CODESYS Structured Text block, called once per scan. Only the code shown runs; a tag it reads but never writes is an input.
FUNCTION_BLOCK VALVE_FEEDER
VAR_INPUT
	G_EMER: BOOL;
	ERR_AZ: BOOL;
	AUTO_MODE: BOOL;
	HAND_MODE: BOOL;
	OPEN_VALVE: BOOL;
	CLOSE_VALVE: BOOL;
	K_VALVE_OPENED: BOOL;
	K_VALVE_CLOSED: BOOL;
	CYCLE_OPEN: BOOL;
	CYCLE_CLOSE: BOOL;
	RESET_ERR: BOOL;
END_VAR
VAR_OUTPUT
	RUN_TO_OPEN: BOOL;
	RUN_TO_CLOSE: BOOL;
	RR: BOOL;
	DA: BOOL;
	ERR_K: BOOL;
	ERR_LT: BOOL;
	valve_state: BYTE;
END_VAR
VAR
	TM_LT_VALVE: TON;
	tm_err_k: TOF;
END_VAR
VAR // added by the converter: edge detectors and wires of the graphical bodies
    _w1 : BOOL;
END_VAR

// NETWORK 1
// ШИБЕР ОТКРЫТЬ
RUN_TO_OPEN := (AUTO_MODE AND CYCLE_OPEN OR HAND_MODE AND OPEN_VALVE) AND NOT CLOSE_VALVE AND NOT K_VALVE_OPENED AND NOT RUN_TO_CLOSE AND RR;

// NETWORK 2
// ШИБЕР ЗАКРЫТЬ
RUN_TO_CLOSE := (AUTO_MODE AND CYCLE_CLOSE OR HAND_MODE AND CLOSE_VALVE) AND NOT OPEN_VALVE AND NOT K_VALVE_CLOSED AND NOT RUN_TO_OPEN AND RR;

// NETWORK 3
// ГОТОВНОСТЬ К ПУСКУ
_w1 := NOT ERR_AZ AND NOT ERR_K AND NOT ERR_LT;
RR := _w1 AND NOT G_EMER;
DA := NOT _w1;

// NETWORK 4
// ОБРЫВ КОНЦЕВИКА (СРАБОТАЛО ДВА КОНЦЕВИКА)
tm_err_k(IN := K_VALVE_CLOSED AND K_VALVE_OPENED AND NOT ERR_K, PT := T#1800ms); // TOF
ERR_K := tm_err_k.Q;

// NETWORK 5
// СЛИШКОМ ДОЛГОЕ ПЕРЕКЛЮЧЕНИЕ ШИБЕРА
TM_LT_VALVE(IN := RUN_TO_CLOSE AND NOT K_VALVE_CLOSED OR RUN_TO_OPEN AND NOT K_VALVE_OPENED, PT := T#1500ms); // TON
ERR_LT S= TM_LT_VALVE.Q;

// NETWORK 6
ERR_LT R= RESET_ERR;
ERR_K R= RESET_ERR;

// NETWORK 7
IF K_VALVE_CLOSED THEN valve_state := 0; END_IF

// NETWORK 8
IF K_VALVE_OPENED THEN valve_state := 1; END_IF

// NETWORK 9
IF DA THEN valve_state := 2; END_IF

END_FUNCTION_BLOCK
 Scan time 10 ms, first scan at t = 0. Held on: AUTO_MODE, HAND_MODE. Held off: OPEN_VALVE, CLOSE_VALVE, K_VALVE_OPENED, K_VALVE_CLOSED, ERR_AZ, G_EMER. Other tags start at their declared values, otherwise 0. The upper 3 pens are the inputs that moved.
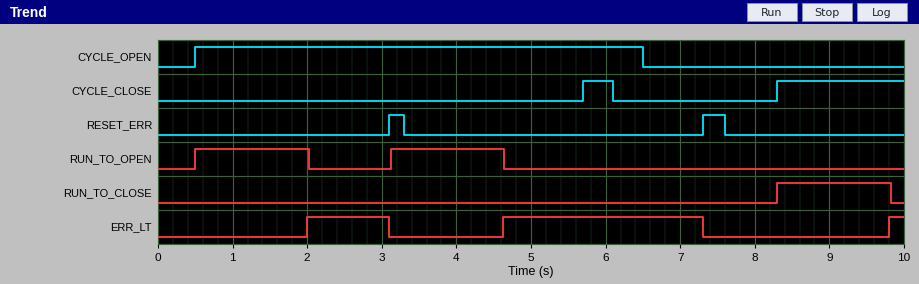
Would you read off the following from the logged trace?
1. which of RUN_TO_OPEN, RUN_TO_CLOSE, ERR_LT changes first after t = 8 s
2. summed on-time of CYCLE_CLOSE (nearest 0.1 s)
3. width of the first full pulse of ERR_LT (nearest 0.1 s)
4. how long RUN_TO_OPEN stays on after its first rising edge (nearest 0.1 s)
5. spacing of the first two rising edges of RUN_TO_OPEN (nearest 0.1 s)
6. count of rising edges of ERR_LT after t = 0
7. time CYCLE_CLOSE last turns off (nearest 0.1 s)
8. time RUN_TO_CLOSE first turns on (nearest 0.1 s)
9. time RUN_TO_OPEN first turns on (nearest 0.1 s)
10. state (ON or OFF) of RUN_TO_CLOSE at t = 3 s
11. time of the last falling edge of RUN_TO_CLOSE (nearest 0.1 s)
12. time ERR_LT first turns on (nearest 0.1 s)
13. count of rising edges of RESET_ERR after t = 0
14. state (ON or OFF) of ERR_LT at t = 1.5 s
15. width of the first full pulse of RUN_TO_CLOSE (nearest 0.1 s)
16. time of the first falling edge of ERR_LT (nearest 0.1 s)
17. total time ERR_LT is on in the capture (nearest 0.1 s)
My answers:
RUN_TO_CLOSE
2.1 s
1.1 s
1.5 s
2.6 s
3
6.1 s
8.3 s
0.5 s
OFF
9.8 s
2.0 s
2
OFF
1.5 s
3.1 s
4.0 s
